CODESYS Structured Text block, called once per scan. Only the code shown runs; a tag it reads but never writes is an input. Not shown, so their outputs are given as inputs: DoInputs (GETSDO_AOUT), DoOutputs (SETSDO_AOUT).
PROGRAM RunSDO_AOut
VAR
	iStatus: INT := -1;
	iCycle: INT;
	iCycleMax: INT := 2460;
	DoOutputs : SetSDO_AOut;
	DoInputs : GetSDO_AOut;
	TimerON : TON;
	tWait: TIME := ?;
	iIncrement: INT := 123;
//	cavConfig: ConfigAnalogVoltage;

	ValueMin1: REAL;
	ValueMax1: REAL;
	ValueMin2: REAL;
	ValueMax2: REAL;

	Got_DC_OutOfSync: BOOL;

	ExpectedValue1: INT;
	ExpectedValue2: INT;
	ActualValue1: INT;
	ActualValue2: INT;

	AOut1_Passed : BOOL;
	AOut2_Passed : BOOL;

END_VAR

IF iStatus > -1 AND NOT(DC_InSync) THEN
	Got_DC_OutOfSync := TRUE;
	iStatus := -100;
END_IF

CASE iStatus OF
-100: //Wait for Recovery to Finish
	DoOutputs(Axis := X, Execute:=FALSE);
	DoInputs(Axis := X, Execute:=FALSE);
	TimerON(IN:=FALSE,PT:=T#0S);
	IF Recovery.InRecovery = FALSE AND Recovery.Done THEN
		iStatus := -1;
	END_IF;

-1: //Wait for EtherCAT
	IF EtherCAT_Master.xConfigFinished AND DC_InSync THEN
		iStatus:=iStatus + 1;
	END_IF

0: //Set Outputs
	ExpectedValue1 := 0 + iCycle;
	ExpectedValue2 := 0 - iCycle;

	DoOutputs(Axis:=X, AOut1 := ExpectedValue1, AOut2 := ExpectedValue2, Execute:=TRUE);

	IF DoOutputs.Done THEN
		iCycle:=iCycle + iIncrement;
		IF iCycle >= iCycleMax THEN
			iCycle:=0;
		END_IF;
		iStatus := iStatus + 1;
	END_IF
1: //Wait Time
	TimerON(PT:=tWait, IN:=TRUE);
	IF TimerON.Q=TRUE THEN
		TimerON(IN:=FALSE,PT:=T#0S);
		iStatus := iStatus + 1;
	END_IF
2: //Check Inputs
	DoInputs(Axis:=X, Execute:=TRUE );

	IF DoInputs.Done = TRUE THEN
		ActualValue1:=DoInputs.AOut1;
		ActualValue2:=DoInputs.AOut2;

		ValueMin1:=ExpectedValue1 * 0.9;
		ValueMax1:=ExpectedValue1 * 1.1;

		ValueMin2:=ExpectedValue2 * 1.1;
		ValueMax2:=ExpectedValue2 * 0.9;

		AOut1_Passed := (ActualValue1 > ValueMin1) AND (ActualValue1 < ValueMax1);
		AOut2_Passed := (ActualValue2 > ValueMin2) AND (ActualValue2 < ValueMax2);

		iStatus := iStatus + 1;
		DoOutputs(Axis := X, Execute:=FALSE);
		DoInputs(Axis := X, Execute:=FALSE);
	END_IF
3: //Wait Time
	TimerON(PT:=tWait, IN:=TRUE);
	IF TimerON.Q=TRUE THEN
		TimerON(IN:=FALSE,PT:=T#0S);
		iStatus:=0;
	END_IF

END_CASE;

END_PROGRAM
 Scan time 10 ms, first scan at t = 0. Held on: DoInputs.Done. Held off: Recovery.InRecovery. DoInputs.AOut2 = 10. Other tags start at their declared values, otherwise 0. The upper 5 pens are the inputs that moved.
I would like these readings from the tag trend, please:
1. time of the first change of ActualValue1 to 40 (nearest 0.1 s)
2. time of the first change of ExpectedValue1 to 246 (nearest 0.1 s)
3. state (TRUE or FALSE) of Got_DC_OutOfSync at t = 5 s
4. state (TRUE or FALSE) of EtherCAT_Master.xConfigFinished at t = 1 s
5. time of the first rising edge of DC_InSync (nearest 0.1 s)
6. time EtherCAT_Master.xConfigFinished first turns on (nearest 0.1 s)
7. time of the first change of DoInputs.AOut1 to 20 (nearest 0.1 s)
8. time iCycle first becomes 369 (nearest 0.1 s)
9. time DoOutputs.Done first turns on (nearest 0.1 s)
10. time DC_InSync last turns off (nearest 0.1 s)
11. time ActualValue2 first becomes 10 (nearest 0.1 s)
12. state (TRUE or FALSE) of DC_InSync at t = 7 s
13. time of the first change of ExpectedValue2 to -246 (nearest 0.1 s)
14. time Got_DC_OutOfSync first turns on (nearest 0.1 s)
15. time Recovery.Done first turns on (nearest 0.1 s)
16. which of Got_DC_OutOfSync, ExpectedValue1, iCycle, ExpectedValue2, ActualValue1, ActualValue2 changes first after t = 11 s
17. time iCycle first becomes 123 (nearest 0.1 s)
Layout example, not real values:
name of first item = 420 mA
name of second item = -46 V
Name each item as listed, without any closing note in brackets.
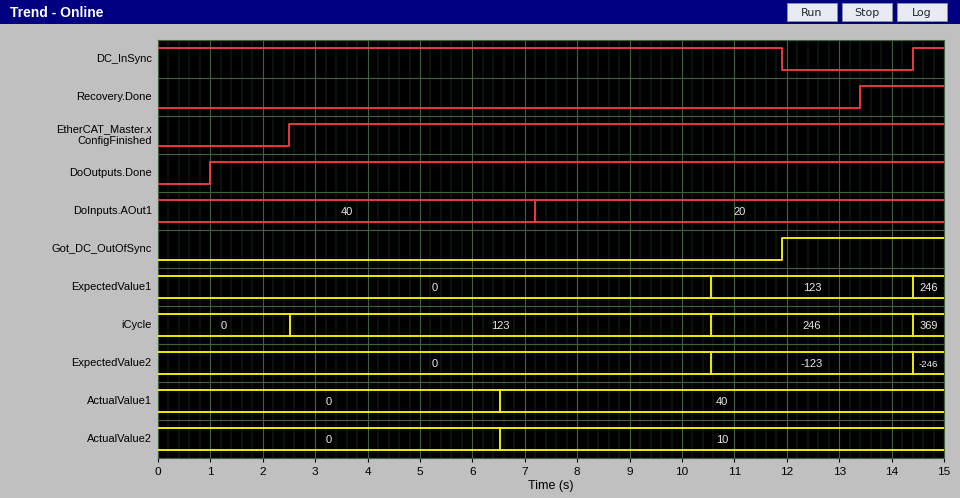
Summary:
time of the first change of ActualValue1 to 40 = 6.5 s
time of the first change of ExpectedValue1 to 246 = 14.4 s
state (TRUE or FALSE) of Got_DC_OutOfSync at t = 5 s = FALSE
state (TRUE or FALSE) of EtherCAT_Master.xConfigFinished at t = 1 s = FALSE
time of the first rising edge of DC_InSync = 14.4 s
time EtherCAT_Master.xConfigFinished first turns on = 2.5 s
time of the first change of DoInputs.AOut1 to 20 = 7.2 s
time iCycle first becomes 369 = 14.4 s
time DoOutputs.Done first turns on = 1.0 s
time DC_InSync last turns off = 11.9 s
time ActualValue2 first becomes 10 = 6.5 s
state (TRUE or FALSE) of DC_InSync at t = 7 s = TRUE
time of the first change of ExpectedValue2 to -246 = 14.4 s
time Got_DC_OutOfSync first turns on = 11.9 s
time Recovery.Done first turns on = 13.4 s
which of Got_DC_OutOfSync, ExpectedValue1, iCycle, ExpectedValue2, ActualValue1, ActualValue2 changes first after t = 11 s = Got_DC_OutOfSync
time iCycle first becomes 123 = 2.5 s
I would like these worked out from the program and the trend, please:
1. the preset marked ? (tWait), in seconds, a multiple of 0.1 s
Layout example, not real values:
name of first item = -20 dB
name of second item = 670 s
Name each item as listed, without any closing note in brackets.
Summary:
the preset marked ? (tWait), in seconds, a multiple of 0.1 s = 4.0 s
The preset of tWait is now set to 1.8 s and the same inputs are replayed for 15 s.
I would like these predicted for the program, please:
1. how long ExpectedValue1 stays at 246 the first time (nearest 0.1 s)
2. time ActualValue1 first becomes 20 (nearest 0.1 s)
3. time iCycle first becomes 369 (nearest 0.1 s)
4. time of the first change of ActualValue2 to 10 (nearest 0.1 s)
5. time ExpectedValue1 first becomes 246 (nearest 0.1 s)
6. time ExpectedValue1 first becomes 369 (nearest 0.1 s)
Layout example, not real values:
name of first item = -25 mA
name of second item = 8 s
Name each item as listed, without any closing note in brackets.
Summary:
how long ExpectedValue1 stays at 246 the first time = 4.6 s
time ActualValue1 first becomes 20 = 8.0 s
time iCycle first becomes 369 = 9.8 s
time of the first change of ActualValue2 to 10 = 4.3 s
time ExpectedValue1 first becomes 246 = 9.8 s
time ExpectedValue1 first becomes 369 = 14.4 s
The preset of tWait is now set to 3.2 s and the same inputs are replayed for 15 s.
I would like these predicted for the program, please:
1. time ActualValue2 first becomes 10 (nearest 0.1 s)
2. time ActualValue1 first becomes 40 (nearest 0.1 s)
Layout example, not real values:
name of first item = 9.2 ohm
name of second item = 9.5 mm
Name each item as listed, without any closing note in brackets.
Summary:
time ActualValue2 first becomes 10 = 5.7 s
time ActualValue1 first becomes 40 = 5.7 s
